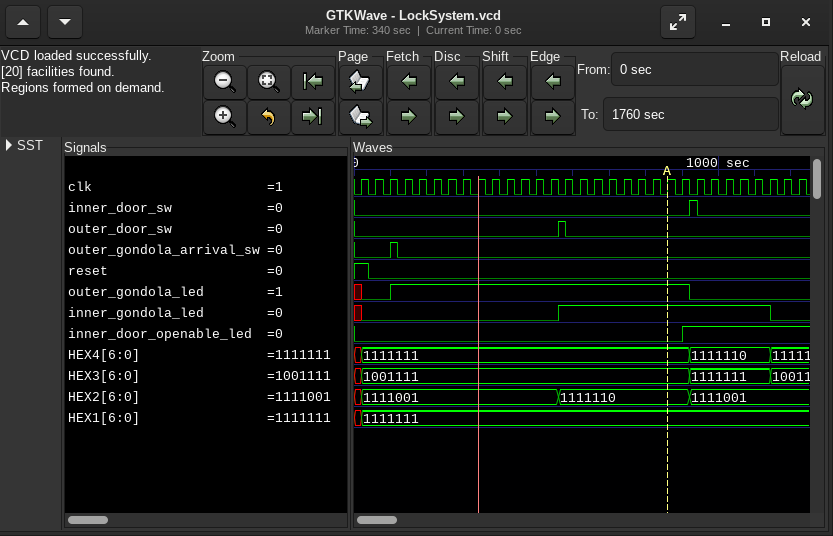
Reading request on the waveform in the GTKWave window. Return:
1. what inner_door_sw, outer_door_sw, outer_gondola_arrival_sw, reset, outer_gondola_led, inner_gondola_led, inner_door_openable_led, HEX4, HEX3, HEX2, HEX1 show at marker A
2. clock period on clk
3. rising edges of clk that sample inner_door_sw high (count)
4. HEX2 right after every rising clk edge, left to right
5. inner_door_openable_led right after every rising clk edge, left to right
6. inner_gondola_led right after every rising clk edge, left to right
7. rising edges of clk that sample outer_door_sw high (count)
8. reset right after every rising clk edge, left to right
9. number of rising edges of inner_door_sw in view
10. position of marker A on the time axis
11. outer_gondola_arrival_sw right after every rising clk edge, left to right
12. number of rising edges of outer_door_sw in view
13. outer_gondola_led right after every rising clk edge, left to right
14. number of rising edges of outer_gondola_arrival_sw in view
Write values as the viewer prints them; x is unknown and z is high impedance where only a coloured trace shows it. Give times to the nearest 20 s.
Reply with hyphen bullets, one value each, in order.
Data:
- inner_door_sw=0, outer_door_sw=0, outer_gondola_arrival_sw=0, reset=0, outer_gondola_led=1, inner_gondola_led=1, inner_door_openable_led=0, HEX4=1111111, HEX3=1001111, HEX2=1111110, HEX1=1111111
- 40 s
- 1
- 1111001, 1111001, 1111001, 1111001, 1111001, 1111001, 1111001, 1111001, 1111001, 1111001, 1111001, 1111001, 1111001, 1111001, 1111110, 1111110, 1111110, 1111110, 1111110, 1111110, 1111110, 1111110, 1111110, 1111001, 1111001, 1111001, 1111001, 1111001, 1111001, 1111001, 1111001
- 0 0 0 0 0 0 0 0 0 0 0 0 0 0 0 0 0 0 0 0 0 0 1 1 1 1 1 1 1 1 1
- 0 0 0 0 0 0 0 0 0 0 0 0 0 0 1 1 1 1 1 1 1 1 1 1 1 1 1 1 0 0 0
- 1
- 1 0 0 0 0 0 0 0 0 0 0 0 0 0 0 0 0 0 0 0 0 0 0 0 0 0 0 0 0 0 0
- 1
- 860 s
- 0 0 1 0 0 0 0 0 0 0 0 0 0 0 0 0 0 0 0 0 0 0 0 0 0 0 0 0 0 0 0
- 1
- 0 0 1 1 1 1 1 1 1 1 1 1 1 1 1 1 1 1 1 1 1 1 1 0 0 0 0 0 0 0 0
- 1
